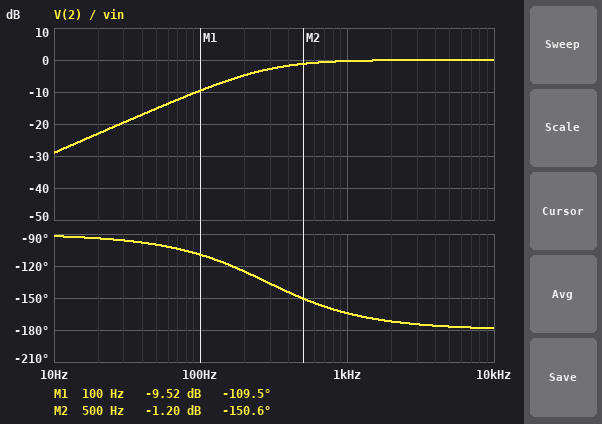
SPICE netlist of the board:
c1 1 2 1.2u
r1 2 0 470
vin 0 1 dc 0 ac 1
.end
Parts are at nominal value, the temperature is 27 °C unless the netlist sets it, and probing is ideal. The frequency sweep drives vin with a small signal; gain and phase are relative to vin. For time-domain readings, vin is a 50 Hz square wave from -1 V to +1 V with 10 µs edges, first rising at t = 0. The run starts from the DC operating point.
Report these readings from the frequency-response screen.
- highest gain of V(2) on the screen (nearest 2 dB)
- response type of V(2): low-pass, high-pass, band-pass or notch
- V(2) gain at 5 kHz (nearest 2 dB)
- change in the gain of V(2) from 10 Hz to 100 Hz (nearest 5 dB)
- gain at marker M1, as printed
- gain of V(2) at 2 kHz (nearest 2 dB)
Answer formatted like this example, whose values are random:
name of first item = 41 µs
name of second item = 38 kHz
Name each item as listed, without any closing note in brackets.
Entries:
highest gain of V(2) on the screen = 0 dB
response type of V(2): low-pass, high-pass, band-pass or notch = high-pass
V(2) gain at 5 kHz = 0 dB
change in the gain of V(2) from 10 Hz to 100 Hz = 20 dB
gain at marker M1, as printed = -9.52 dB
gain of V(2) at 2 kHz = 0 dB
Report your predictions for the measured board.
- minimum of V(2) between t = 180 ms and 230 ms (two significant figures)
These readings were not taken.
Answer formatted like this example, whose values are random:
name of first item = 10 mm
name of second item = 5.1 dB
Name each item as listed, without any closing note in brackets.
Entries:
minimum of V(2) between t = 180 ms and 230 ms = -2.0 V
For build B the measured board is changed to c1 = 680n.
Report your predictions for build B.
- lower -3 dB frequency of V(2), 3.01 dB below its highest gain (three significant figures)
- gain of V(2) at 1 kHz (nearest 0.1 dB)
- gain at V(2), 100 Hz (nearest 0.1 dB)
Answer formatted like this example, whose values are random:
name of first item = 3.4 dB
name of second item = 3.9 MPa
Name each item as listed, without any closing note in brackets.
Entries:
lower -3 dB frequency of V(2), 3.01 dB below its highest gain = 498 Hz
gain of V(2) at 1 kHz = -1.0 dB
gain at V(2), 100 Hz = -14.1 dB
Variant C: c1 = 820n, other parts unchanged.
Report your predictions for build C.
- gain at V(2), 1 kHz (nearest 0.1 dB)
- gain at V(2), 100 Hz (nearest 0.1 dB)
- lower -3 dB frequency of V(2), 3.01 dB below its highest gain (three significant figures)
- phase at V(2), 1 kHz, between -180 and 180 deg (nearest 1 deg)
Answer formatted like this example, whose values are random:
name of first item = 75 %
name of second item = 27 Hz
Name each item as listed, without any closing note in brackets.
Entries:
gain at V(2), 1 kHz = -0.7 dB
gain at V(2), 100 Hz = -12.6 dB
lower -3 dB frequency of V(2), 3.01 dB below its highest gain = 413 Hz
phase at V(2), 1 kHz, between -180 and 180 deg = -158 deg
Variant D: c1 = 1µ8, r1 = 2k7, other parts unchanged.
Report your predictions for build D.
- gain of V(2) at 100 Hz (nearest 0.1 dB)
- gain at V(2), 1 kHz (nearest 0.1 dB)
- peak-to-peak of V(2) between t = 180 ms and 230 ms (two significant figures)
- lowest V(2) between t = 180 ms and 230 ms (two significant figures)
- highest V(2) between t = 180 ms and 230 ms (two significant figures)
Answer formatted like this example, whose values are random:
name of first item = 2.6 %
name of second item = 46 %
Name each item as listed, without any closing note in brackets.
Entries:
gain of V(2) at 100 Hz = -0.4 dB
gain at V(2), 1 kHz = 0 dB
peak-to-peak of V(2) between t = 180 ms and 230 ms = 3.5 V
lowest V(2) between t = 180 ms and 230 ms = -1.8 V
highest V(2) between t = 180 ms and 230 ms = 1.8 V
